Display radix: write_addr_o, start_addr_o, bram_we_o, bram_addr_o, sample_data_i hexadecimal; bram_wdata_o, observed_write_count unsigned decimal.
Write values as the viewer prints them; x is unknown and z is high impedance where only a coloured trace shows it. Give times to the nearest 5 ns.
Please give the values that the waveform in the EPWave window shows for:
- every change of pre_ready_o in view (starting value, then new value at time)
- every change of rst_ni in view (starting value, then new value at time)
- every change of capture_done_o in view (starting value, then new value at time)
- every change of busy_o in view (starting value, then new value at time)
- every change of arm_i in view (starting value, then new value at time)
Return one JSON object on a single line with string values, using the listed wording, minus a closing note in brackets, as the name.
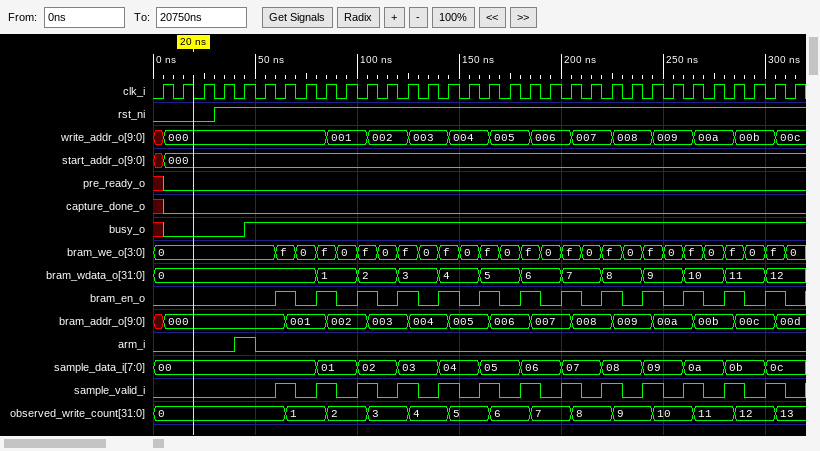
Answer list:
{"every change of pre_ready_o in view": "x, 0 at 5 ns", "every change of rst_ni in view": "0, 1 at 30 ns", "every change of capture_done_o in view": "x, 0 at 5 ns", "every change of busy_o in view": "x, 0 at 5 ns, 1 at 45 ns", "every change of arm_i in view": "0, 1 at 40 ns, 0 at 50 ns"}
